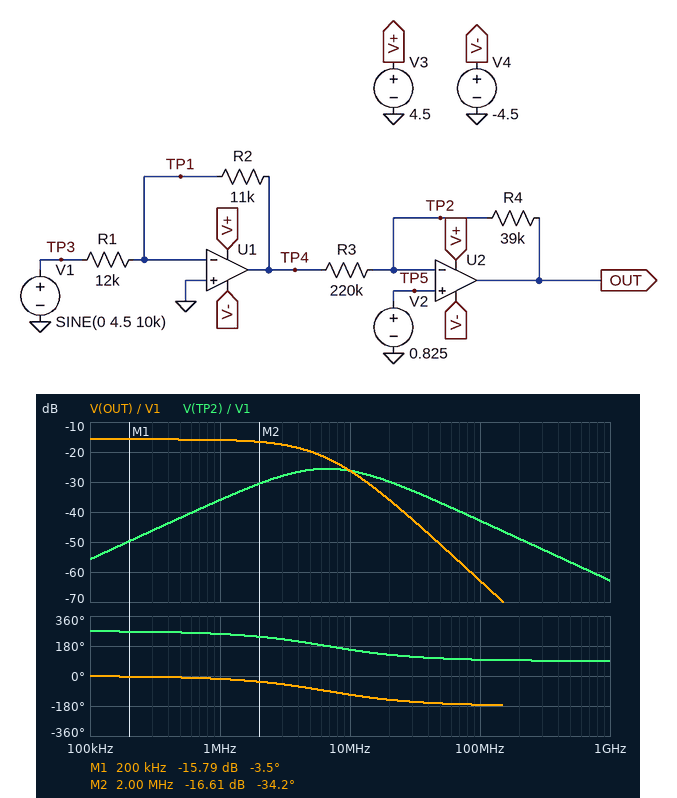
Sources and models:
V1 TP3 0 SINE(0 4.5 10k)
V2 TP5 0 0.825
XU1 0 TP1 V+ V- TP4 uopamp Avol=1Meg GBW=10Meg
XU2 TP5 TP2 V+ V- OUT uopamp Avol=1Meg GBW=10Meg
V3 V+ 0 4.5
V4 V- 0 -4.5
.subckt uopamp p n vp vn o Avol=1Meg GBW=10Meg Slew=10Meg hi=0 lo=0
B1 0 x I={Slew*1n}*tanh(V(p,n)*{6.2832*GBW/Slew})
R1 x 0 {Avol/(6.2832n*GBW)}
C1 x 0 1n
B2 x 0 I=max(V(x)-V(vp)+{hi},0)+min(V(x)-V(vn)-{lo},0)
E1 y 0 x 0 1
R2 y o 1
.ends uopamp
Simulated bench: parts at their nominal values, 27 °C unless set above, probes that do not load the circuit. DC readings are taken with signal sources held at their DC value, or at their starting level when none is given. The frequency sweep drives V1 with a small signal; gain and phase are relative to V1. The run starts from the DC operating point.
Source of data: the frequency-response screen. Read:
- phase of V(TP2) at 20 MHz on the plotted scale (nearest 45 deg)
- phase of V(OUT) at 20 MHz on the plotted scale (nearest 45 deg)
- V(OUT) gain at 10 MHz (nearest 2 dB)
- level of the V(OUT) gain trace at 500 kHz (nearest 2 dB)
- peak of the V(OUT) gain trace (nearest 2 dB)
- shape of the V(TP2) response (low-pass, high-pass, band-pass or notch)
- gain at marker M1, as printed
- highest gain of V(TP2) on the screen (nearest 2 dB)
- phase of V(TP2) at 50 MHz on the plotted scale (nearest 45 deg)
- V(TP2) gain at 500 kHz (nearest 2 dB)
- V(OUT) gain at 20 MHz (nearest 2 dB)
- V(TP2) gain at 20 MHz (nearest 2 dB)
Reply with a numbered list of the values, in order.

1. 135 deg
2. -135 deg
3. -26 dB
4. -16 dB
5. -16 dB
6. band-pass
7. -15.79 dB
8. -26 dB
9. 90 deg
10. -42 dB
11. -36 dB
12. -30 dB
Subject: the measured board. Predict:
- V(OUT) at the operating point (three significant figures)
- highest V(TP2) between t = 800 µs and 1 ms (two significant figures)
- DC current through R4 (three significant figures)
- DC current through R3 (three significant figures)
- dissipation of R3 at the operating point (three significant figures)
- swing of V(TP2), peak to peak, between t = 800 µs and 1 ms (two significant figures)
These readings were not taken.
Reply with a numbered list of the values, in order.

1. 971 mV
2. 830 mV
3. 3.75 µA
4. 3.75 µA
5. 3.09 µW
6. 1.5 mV
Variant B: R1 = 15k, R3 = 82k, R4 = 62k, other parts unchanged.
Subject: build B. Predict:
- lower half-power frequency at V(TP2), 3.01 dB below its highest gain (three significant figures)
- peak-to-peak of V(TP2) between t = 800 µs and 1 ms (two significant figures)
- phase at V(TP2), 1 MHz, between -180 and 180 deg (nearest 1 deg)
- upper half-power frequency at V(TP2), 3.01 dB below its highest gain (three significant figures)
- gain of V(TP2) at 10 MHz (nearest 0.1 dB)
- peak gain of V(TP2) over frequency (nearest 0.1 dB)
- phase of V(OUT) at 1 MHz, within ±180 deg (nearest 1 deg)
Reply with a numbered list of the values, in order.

1. 2.37 MHz
2. 5.0 mV
3. -110 deg
4. 13.8 MHz
5. -17.3 dB
6. -16.0 dB
7. -20 deg
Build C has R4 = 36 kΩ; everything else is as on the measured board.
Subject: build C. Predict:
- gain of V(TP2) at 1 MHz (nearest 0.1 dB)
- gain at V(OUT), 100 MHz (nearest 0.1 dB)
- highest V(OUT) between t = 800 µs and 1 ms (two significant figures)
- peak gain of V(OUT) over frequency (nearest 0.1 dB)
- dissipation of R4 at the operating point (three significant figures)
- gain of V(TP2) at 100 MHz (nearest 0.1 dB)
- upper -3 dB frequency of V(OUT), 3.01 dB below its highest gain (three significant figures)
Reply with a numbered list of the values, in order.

1. -36.7 dB
2. -63.5 dB
3. 1.6 V
4. -16.5 dB
5. 506 nW
6. -43.5 dB
7. 4.13 MHz
